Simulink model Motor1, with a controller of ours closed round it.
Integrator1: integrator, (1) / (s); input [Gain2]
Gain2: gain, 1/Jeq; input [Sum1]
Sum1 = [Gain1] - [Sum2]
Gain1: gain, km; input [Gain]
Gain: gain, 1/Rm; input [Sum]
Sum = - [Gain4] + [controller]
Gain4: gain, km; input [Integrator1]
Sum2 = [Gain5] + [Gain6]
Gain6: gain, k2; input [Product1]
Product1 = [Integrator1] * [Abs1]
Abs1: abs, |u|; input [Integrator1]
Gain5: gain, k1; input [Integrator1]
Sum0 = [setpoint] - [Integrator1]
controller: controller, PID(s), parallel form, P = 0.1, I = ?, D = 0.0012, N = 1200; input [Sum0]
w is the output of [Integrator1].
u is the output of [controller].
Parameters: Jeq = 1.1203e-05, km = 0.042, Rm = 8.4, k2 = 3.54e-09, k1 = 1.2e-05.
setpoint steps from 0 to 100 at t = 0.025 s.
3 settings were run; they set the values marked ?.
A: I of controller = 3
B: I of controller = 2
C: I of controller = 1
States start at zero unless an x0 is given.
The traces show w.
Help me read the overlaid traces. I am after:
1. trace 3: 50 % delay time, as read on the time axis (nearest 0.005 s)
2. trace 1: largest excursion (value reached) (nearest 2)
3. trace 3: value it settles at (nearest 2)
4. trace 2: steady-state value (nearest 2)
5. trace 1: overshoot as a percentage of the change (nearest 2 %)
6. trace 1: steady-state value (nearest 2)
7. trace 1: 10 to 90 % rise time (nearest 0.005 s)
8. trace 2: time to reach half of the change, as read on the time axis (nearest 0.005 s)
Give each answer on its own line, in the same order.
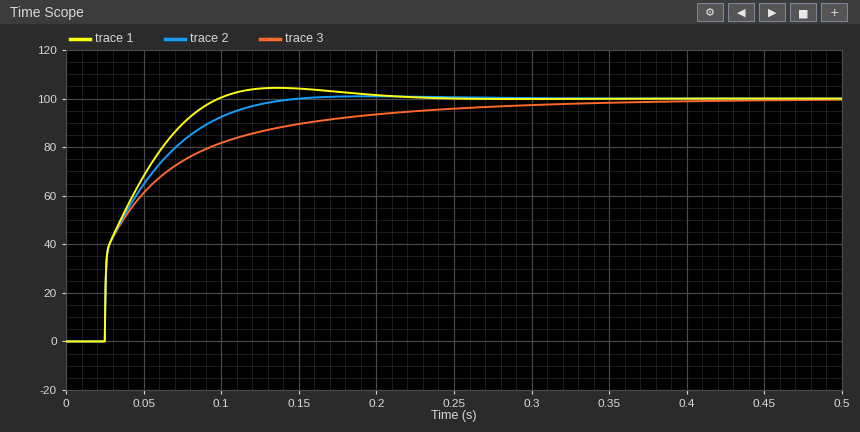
0.035 s
104
100
100
4 %
100
0.050 s
0.035 s
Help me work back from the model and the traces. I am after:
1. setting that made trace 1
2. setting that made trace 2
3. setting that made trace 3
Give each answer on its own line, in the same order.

A
B
C
